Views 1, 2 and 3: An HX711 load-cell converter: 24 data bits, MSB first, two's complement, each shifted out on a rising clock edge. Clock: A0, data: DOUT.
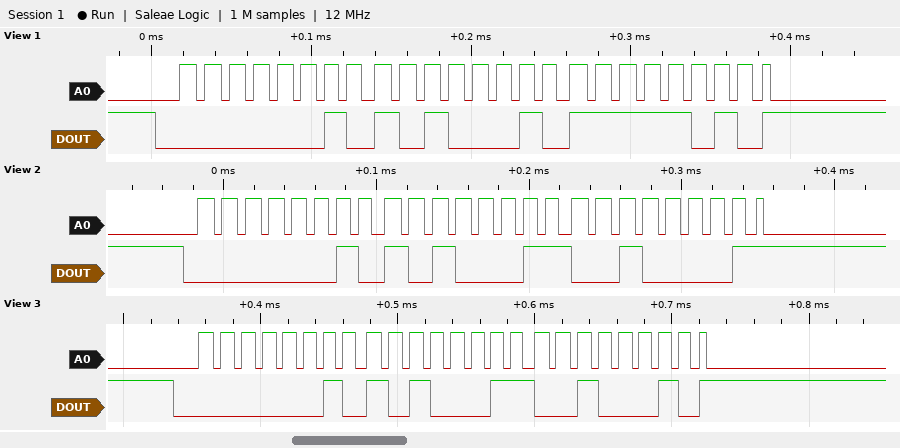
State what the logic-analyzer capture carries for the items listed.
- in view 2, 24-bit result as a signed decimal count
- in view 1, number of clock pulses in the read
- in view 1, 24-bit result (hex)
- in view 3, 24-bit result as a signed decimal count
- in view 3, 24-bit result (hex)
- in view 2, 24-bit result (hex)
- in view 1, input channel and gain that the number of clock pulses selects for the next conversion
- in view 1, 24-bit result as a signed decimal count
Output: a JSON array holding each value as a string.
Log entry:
["172833", "25", "0x02A2FA", "172834", "0x02A322", "0x02A321", "channel A, gain 128", "172794"]
